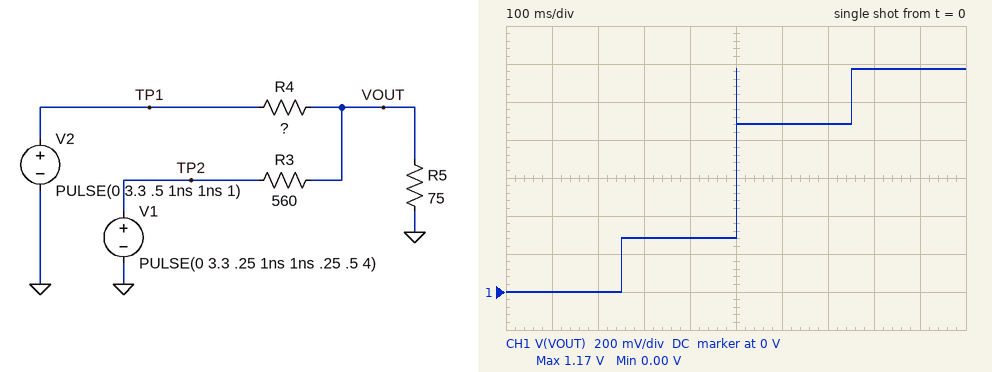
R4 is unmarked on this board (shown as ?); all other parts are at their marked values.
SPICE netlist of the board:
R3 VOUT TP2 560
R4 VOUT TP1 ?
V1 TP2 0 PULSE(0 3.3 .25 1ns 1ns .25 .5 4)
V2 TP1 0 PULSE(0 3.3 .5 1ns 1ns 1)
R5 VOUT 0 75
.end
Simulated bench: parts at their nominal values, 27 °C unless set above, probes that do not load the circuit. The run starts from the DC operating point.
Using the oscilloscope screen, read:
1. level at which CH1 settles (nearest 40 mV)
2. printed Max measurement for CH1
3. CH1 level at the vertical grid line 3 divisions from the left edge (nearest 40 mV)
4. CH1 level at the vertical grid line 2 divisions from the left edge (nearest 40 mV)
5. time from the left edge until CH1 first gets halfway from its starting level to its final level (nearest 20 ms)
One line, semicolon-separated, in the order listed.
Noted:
1.16 V; 1.17 V; 280 mV; 0 V; 500 ms
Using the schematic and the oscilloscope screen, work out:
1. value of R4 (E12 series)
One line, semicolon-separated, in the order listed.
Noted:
180 Ω
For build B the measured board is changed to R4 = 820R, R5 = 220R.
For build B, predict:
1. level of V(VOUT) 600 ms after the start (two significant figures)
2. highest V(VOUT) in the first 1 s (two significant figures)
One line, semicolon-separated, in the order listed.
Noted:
530 mV; 1.3 V
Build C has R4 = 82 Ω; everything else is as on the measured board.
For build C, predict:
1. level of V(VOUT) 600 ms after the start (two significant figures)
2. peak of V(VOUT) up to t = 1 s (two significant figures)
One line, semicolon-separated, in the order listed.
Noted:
1.5 V; 1.7 V
